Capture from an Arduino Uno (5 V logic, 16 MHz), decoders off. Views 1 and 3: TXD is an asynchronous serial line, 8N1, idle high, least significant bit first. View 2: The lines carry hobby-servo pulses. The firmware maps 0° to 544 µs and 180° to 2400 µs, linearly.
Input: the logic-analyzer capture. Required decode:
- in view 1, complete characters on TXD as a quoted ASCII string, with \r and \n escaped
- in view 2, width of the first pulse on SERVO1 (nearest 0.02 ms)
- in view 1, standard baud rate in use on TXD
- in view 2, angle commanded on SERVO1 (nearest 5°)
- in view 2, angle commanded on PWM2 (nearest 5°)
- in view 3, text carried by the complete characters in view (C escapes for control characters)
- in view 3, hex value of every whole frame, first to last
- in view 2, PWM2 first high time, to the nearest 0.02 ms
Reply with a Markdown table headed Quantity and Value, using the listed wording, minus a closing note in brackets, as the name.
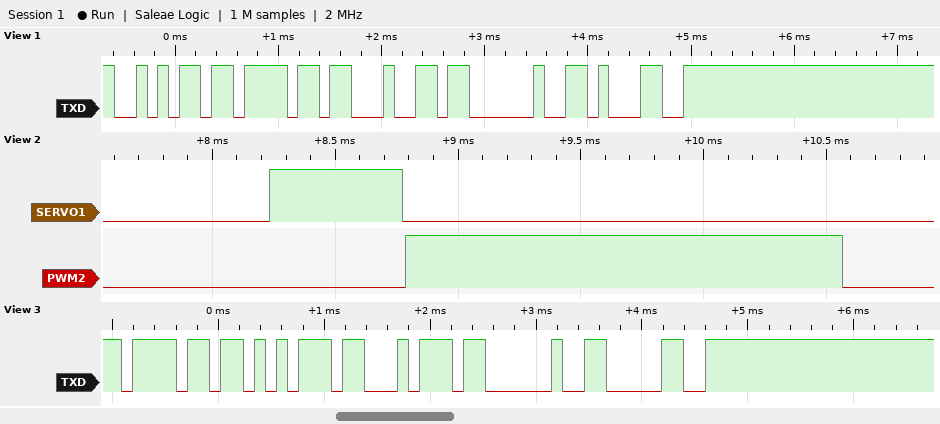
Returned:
| Quantity | Value |
|---|---|
| in view 1, complete characters on TXD as a quoted ASCII string, with \r and \n escaped | "jod 1" |
| in view 2, width of the first pulse on SERVO1 | 0.54 ms |
| in view 1, standard baud rate in use on TXD | 9600 baud |
| in view 2, angle commanded on SERVO1 | 0° |
| in view 2, angle commanded on PWM2 | 120° |
| in view 3, text carried by the complete characters in view | "out 0" |
| in view 3, hex value of every whole frame, first to last | 6F 75 74 20 30 |
| in view 2, PWM2 first high time, to the nearest 0.02 ms | 1.78 ms |
